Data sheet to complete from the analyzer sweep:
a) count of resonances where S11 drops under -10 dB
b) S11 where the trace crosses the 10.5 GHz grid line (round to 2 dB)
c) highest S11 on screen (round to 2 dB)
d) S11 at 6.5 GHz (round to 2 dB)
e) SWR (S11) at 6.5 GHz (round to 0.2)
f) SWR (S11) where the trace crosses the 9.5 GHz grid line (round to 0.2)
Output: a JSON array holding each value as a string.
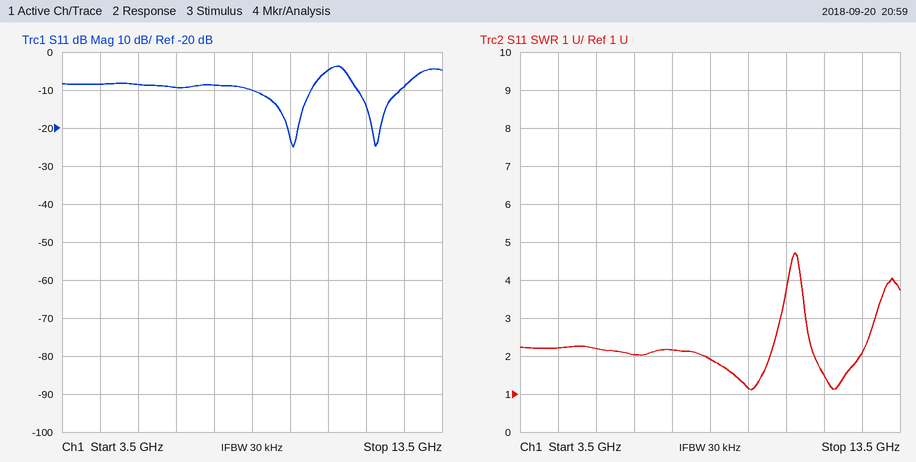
["2", "-4 dB", "-4 dB", "-10 dB", "2.0", "1.2"]
